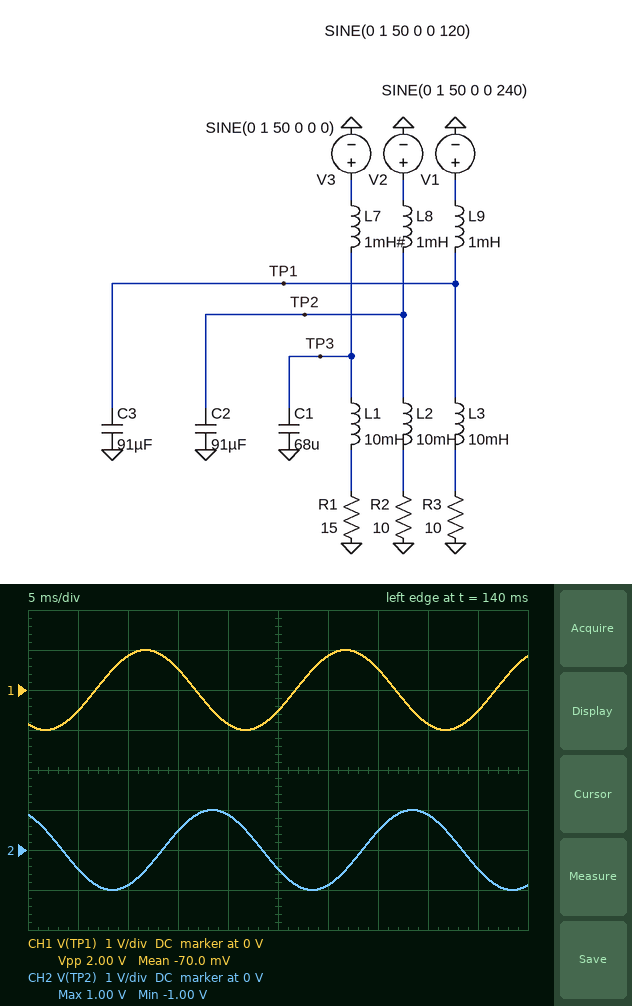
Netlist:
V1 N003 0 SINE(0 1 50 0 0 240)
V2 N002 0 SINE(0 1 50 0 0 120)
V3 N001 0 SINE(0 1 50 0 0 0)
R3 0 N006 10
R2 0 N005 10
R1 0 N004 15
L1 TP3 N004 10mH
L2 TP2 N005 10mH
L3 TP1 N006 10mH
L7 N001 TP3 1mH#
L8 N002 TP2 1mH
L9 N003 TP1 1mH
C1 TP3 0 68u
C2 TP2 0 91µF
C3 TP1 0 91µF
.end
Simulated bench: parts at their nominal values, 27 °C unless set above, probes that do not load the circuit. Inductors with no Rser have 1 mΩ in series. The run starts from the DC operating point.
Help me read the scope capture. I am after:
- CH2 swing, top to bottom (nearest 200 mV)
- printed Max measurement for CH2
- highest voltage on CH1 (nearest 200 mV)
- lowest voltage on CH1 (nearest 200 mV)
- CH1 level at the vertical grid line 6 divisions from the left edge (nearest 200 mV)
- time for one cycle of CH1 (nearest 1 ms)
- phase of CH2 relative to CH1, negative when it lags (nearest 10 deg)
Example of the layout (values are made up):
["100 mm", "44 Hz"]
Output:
["2.0 V", "1.00 V", "1.0 V", "-1.0 V", "800 mV", "20 ms", "-120 deg"]
